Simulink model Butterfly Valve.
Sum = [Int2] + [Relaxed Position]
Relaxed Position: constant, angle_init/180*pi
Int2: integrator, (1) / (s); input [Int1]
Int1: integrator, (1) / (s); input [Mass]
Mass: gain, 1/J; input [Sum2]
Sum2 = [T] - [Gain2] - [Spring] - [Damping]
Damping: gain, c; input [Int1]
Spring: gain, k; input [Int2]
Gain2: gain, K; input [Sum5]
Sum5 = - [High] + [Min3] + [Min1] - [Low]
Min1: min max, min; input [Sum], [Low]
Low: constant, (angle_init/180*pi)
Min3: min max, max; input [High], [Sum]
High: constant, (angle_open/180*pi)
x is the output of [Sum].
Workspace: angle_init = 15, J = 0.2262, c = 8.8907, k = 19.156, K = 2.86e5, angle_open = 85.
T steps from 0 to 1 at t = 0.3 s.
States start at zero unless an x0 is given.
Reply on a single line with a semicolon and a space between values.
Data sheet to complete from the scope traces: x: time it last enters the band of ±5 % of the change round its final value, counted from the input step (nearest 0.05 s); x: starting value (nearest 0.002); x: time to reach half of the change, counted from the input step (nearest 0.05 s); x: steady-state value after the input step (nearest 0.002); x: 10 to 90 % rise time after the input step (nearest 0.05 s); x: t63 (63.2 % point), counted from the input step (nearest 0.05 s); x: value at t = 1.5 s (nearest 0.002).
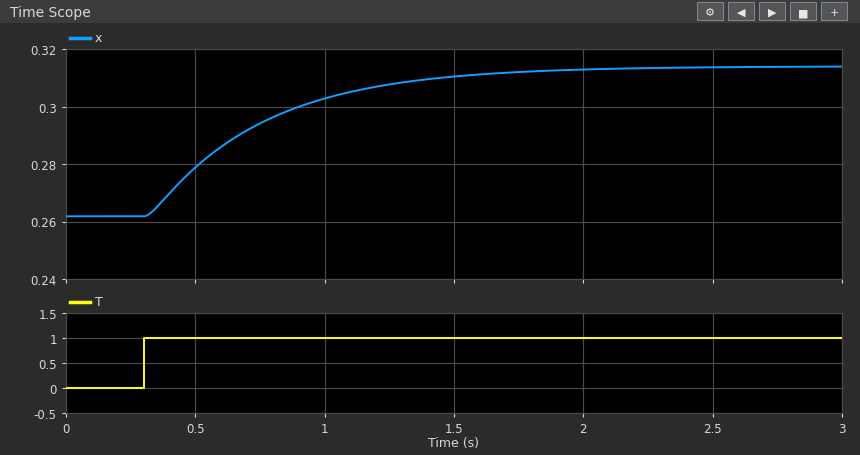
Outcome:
1.35 s; 0.262; 0.35 s; 0.314; 0.95 s; 0.45 s; 0.310
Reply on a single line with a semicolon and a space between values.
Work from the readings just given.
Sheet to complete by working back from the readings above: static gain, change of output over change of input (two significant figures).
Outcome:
0.052
